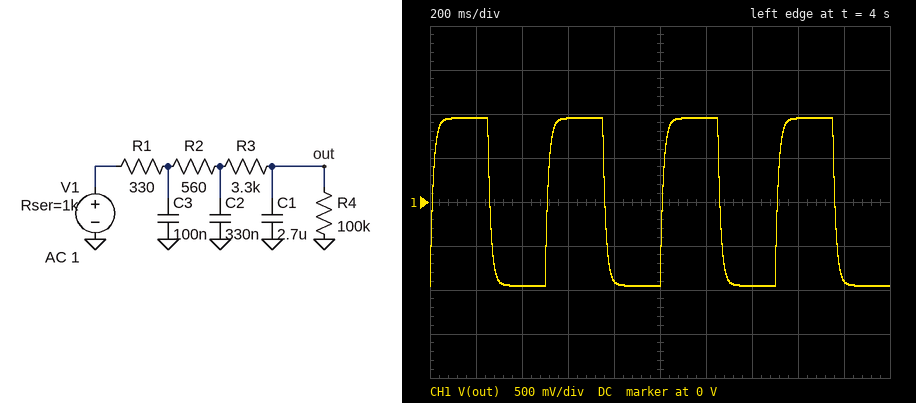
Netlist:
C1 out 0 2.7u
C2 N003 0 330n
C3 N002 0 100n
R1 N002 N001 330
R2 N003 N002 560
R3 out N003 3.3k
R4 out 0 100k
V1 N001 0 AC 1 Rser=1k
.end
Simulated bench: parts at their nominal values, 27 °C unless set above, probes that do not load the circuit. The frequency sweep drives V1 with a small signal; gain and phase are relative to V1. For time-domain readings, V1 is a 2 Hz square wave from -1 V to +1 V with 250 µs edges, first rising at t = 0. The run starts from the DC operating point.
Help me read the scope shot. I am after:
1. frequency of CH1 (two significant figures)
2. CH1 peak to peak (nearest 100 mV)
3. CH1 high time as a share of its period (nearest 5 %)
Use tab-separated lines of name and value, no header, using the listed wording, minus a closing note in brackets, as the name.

frequency of CH1	2.0 Hz
CH1 peak to peak	1.9 V
CH1 high time as a share of its period	50 %
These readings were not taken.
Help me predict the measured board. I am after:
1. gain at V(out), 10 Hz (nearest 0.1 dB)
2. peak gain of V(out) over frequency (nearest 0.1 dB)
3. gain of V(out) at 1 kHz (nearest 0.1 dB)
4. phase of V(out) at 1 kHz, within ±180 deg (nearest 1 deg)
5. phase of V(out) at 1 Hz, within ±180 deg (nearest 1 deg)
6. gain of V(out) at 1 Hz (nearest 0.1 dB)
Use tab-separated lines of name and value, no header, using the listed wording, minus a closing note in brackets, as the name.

gain at V(out), 10 Hz	-2.8 dB
peak gain of V(out) over frequency	-0.4 dB
gain of V(out) at 1 kHz	-48.8 dB
phase of V(out) at 1 kHz, within ±180 deg	-172 deg
phase of V(out) at 1 Hz, within ±180 deg	-5 deg
gain of V(out) at 1 Hz	-0.5 dB
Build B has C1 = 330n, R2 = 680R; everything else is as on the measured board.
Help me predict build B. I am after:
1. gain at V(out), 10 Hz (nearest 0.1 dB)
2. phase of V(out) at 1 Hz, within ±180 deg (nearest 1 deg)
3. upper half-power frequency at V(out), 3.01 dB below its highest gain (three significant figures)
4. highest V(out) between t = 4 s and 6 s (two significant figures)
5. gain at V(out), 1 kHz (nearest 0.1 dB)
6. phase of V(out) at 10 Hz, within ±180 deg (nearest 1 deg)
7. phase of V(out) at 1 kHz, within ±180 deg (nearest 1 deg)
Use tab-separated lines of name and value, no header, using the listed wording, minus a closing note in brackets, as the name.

gain at V(out), 10 Hz	-0.5 dB
phase of V(out) at 1 Hz, within ±180 deg	-1 deg
upper half-power frequency at V(out), 3.01 dB below its highest gain	76.2 Hz
highest V(out) between t = 4 s and 6 s	950 mV
gain at V(out), 1 kHz	-31.2 dB
phase of V(out) at 10 Hz, within ±180 deg	-9 deg
phase of V(out) at 1 kHz, within ±180 deg	-167 deg
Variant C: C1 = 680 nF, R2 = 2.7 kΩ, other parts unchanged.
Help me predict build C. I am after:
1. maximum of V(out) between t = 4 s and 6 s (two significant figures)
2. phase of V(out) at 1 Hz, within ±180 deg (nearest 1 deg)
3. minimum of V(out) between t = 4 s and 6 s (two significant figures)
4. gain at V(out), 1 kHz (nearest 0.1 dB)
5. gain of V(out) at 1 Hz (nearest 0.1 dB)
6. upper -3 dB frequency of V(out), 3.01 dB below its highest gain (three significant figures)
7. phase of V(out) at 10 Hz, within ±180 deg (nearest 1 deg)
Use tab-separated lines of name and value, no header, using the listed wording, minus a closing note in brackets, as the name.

maximum of V(out) between t = 4 s and 6 s	930 mV
phase of V(out) at 1 Hz, within ±180 deg	-2 deg
minimum of V(out) between t = 4 s and 6 s	-930 mV
gain at V(out), 1 kHz	-43.2 dB
gain of V(out) at 1 Hz	-0.6 dB
upper -3 dB frequency of V(out), 3.01 dB below its highest gain	29.0 Hz
phase of V(out) at 10 Hz, within ±180 deg	-21 deg
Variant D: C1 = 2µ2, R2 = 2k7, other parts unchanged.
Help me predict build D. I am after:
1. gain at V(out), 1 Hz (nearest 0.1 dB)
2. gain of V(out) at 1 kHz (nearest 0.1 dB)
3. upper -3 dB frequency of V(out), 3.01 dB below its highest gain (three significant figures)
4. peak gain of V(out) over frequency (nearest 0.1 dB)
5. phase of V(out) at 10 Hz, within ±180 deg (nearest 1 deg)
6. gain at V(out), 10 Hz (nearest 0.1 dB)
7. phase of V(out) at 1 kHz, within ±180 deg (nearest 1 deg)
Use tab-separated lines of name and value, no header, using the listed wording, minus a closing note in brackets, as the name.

gain at V(out), 1 Hz	-0.7 dB
gain of V(out) at 1 kHz	-53.4 dB
upper -3 dB frequency of V(out), 3.01 dB below its highest gain	10.1 Hz
peak gain of V(out) over frequency	-0.6 dB
phase of V(out) at 10 Hz, within ±180 deg	-47 deg
gain at V(out), 10 Hz	-3.6 dB
phase of V(out) at 1 kHz, within ±180 deg	167 deg
